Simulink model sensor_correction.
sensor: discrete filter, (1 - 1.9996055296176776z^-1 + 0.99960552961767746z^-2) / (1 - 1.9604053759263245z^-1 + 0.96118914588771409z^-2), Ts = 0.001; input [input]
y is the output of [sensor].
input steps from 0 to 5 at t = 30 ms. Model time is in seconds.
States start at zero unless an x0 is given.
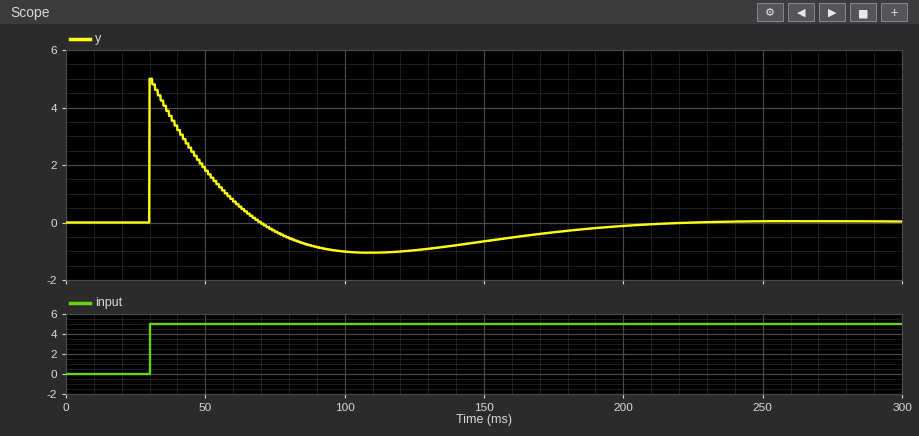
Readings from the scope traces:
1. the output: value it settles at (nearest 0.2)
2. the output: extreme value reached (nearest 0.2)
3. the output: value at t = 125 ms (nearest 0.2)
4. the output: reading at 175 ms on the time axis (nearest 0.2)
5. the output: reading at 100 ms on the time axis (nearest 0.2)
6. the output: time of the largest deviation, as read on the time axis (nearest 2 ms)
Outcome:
0.0
5.0
-1.0
-0.4
-1.0
30 ms
